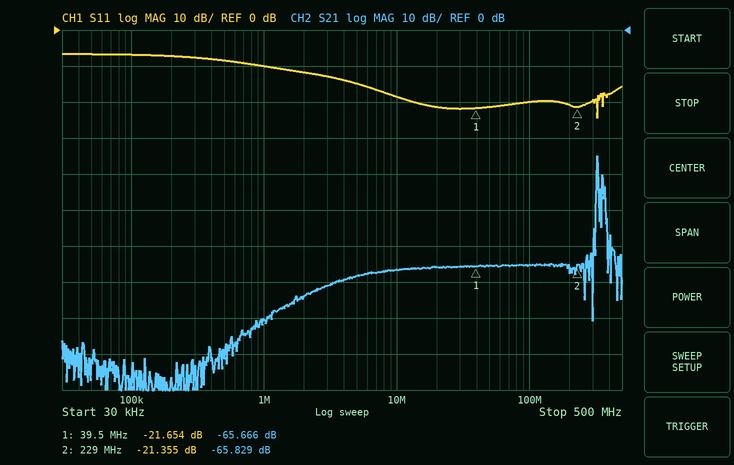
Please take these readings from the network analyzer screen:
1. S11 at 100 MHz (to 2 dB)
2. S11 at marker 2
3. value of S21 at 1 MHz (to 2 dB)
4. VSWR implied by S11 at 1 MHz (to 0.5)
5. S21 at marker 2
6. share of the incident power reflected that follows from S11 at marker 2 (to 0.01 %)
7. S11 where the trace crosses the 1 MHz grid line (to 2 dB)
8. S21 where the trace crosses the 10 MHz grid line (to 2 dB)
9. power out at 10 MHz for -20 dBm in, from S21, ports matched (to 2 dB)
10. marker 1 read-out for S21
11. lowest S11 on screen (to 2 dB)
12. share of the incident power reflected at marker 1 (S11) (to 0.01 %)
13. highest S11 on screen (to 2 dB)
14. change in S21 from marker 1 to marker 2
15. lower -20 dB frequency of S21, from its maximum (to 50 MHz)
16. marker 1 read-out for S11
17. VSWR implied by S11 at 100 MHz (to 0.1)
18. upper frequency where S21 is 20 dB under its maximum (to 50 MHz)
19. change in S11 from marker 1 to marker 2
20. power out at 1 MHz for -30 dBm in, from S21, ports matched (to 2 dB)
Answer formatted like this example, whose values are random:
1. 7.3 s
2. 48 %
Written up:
1. -20 dB
2. -21.355 dB
3. -80 dB
4. 2.0
5. -65.829 dB
6. 0.73 %
7. -10 dB
8. -66 dB
9. -86 dBm
10. -65.666 dB
11. -24 dB
12. 0.68 %
13. -6 dB
14. -0.163 dB
15. 300 MHz
16. -21.654 dB
17. 1.2
18. 400 MHz
19. 0.299 dB
20. -110 dBm
